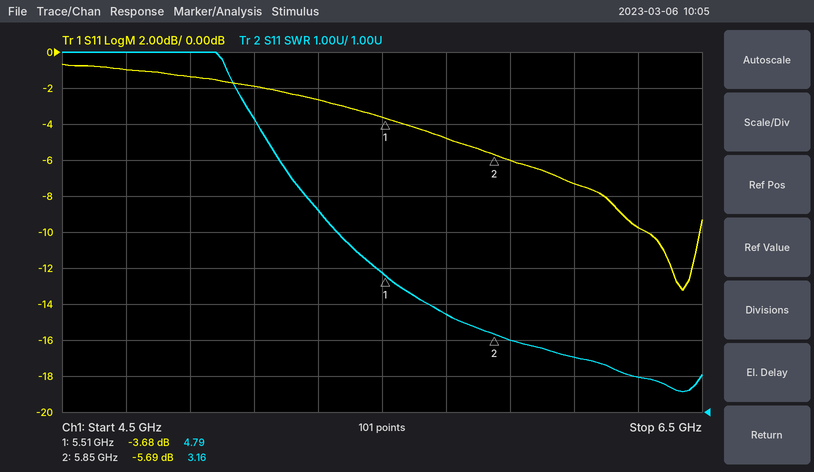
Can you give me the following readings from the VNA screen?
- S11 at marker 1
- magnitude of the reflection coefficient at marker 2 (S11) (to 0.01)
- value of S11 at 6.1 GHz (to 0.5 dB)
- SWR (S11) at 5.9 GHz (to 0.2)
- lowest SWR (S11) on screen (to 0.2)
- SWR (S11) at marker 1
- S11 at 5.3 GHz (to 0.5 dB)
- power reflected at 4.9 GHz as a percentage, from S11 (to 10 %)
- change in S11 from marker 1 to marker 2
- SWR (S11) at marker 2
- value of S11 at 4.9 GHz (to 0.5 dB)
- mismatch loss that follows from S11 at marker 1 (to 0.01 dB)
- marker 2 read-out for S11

-3.68 dB
0.52
-7.5 dB
3.0
1.6
4.79
-2.5 dB
70 %
-2.01 dB
3.16
-1.5 dB
2.43 dB
-5.69 dB
